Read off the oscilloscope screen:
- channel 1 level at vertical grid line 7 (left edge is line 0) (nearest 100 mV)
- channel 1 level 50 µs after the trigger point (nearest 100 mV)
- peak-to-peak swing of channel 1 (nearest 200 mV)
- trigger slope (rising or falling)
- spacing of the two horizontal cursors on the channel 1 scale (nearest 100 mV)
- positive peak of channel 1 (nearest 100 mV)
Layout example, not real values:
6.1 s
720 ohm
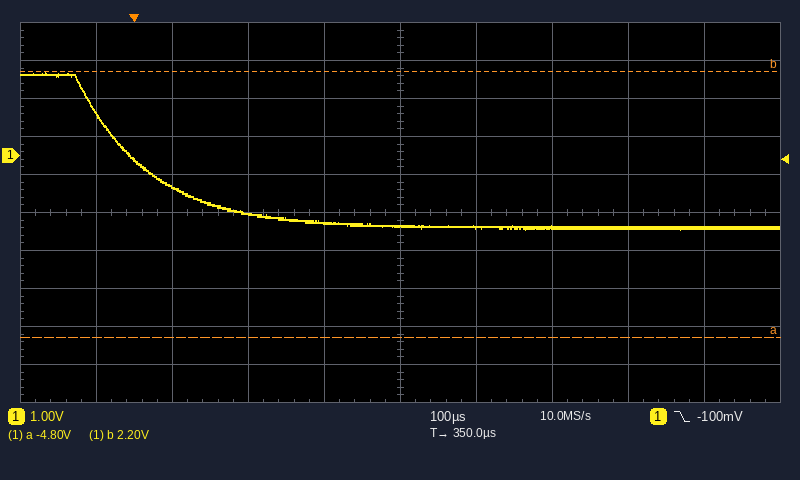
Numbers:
-1.9 V
-800 mV
4.2 V
falling
7.0 V
2.2 V
